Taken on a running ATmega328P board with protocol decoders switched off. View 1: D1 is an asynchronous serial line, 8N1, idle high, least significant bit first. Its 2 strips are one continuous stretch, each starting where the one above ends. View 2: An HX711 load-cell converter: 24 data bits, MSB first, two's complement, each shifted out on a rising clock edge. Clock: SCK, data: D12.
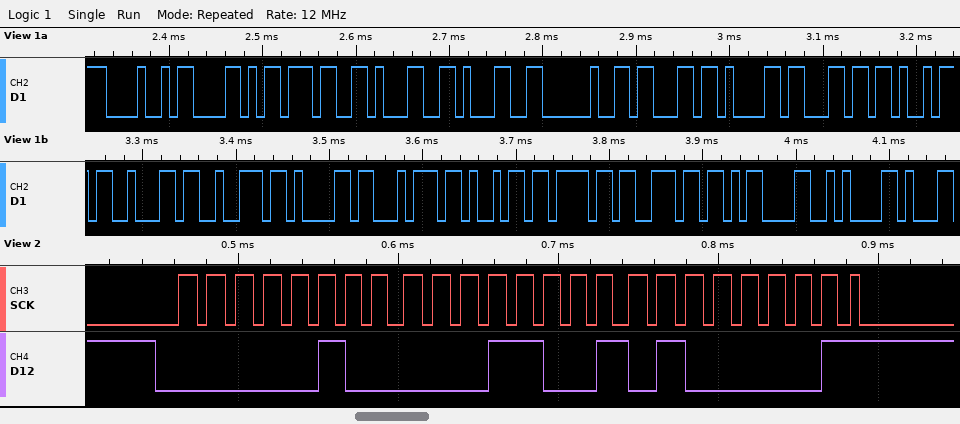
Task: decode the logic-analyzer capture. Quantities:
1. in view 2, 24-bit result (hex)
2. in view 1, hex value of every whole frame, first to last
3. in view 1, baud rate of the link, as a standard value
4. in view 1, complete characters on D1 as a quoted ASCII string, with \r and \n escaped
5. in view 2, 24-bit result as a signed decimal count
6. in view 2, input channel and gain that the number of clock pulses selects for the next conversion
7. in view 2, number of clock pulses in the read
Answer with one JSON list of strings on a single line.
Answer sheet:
["0x041941", "48 58 37 31 31 20 63 61 6C 69 62 72 61 74 69 6F 6E 0D 0A", "115200 baud", "\"HX711 calibration\\r\\n\"", "268609", "channel A, gain 128", "25"]
